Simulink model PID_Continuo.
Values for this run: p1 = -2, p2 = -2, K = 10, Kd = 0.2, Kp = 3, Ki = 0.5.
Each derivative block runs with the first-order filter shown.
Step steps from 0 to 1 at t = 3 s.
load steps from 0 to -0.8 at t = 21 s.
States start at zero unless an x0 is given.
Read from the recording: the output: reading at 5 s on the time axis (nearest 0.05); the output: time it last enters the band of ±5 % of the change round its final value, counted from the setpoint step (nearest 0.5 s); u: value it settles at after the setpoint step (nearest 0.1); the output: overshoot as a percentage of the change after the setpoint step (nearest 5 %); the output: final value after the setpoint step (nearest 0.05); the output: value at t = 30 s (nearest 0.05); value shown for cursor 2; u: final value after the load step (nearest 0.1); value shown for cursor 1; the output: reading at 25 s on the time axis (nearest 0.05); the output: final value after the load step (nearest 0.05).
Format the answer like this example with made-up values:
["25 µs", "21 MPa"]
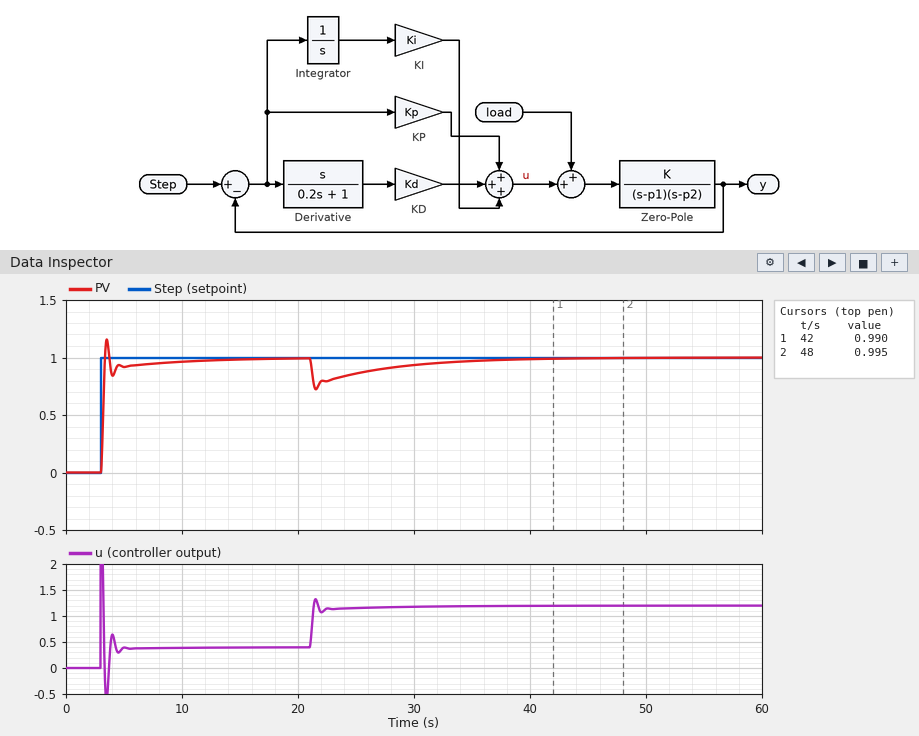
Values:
["0.90", "5.0 s", "0.4", "15 %", "1.00", "0.95", "0.995", "1.2", "0.990", "0.85", "1.00"]
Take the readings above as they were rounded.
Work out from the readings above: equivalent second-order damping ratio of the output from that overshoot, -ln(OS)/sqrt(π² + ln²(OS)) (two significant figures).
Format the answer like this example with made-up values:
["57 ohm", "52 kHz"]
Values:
["0.52"]
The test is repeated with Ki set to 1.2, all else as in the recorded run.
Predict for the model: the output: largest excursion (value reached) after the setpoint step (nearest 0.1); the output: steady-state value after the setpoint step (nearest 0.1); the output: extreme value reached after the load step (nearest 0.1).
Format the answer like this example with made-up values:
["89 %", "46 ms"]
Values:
["1.2", "1.0", "0.7"]
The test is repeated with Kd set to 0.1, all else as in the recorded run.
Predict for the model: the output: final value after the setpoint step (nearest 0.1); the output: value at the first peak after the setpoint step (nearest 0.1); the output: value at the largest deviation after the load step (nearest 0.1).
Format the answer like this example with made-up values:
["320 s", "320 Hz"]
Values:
["1.0", "1.2", "0.7"]
